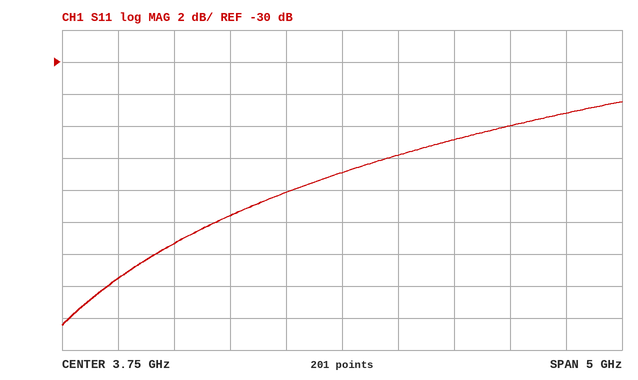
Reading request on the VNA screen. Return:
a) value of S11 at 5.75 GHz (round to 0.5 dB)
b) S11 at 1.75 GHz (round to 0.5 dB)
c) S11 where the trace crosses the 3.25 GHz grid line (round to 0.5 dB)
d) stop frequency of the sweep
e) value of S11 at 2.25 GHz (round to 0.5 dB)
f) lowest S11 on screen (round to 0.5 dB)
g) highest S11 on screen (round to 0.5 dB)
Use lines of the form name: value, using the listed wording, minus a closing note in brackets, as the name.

value of S11 at 5.75 GHz: -33.0 dB
S11 at 1.75 GHz: -43.5 dB
S11 where the trace crosses the 3.25 GHz grid line: -38.0 dB
stop frequency of the sweep: 6.25 GHz
value of S11 at 2.25 GHz: -41.5 dB
lowest S11 on screen: -46.5 dB
highest S11 on screen: -32.5 dB
